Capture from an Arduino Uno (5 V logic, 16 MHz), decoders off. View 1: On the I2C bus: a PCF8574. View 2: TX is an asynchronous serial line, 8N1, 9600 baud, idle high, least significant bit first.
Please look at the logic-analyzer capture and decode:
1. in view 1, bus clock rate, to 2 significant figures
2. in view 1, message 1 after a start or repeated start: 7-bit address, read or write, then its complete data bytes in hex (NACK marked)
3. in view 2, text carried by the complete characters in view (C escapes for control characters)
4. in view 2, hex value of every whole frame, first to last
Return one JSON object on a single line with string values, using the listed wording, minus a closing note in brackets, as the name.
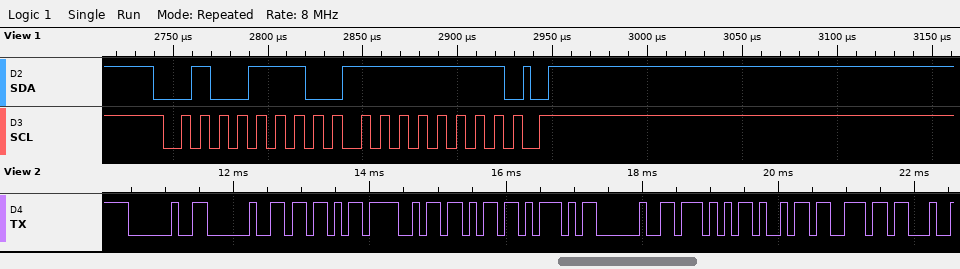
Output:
{"in view 1, bus clock rate, to 2 significant figures": "100 kHz", "in view 1, message 1 after a start or repeated start: 7-bit address, read or write, then its complete data bytes in hex": "0x27 write: FF", "in view 2, text carried by the complete characters in view": "\"  [Ok] Win\"", "in view 2, hex value of every whole frame, first to last": "20 20 5B 4F 6B 5D 20 57 69 6E"}
